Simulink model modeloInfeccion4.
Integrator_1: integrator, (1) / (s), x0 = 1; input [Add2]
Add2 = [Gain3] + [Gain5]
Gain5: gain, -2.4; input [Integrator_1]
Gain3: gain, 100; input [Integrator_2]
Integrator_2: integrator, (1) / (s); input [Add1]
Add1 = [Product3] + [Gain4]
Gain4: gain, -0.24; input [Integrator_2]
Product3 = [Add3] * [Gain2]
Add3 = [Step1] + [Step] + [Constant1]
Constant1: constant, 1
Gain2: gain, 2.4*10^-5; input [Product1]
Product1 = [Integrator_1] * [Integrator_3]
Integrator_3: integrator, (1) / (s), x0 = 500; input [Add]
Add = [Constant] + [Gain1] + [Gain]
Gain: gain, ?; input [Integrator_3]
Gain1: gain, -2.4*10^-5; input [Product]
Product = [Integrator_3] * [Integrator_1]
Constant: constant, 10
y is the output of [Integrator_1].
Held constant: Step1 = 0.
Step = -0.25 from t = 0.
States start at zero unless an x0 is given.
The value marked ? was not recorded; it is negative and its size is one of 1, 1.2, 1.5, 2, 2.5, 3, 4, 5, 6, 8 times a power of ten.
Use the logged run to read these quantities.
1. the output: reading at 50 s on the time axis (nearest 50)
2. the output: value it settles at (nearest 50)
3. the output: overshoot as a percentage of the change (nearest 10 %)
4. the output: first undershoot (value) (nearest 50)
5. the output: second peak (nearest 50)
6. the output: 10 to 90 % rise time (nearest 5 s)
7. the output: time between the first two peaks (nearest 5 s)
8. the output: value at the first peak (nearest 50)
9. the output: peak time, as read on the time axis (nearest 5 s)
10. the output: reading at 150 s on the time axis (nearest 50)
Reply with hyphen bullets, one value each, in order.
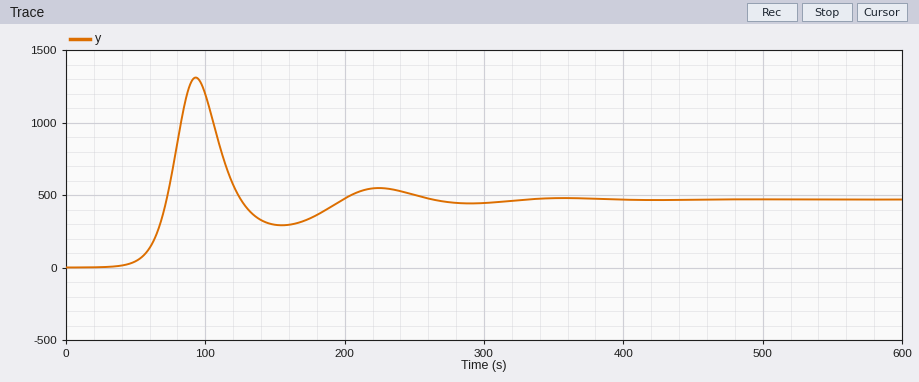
- 50
- 450
- 180 %
- 300
- 550
- 20 s
- 130 s
- 1300
- 95 s
- 300
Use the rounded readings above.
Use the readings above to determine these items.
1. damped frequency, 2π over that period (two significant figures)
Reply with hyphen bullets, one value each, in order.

- 0.048 rad/s
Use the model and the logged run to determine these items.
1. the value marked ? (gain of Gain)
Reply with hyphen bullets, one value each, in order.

- -0.02
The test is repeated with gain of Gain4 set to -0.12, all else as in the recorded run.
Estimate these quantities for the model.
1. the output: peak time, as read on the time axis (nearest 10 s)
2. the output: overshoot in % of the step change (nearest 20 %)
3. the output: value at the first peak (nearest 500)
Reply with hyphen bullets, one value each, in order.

- 60 s
- 200 %
- 5500
